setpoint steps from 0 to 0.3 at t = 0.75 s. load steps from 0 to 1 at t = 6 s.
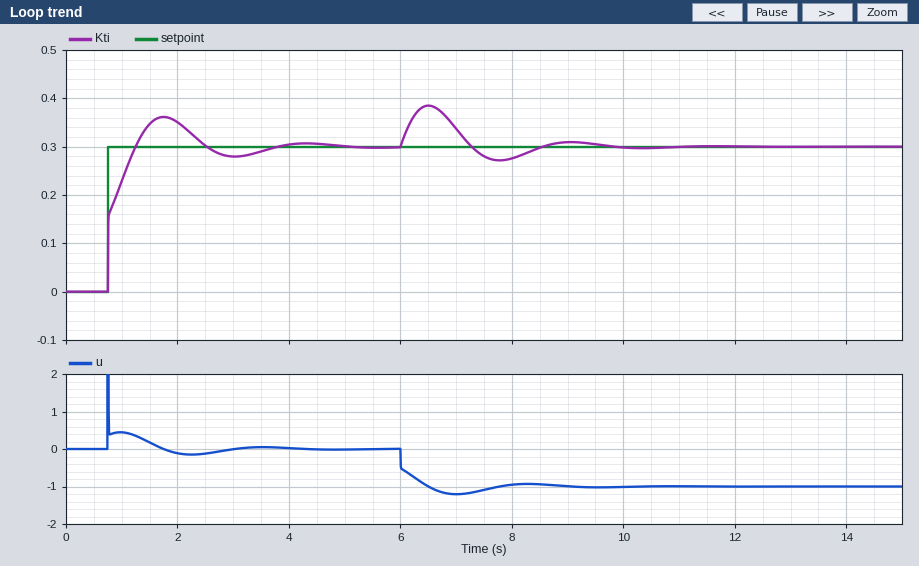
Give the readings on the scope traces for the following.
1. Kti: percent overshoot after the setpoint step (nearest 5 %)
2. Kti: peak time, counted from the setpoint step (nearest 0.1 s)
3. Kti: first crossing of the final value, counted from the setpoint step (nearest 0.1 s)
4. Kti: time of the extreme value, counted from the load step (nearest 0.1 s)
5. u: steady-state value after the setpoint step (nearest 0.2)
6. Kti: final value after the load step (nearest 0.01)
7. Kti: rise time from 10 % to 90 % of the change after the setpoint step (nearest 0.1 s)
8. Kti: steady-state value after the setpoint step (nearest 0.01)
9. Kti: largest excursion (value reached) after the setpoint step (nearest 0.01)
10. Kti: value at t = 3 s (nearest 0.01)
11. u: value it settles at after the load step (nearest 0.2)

20 %
1.0 s
0.5 s
0.5 s
0.0
0.30
0.4 s
0.30
0.36
0.28
-1.0
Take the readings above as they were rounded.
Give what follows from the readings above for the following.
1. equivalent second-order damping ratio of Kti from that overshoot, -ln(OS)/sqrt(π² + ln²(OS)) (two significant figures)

0.46
